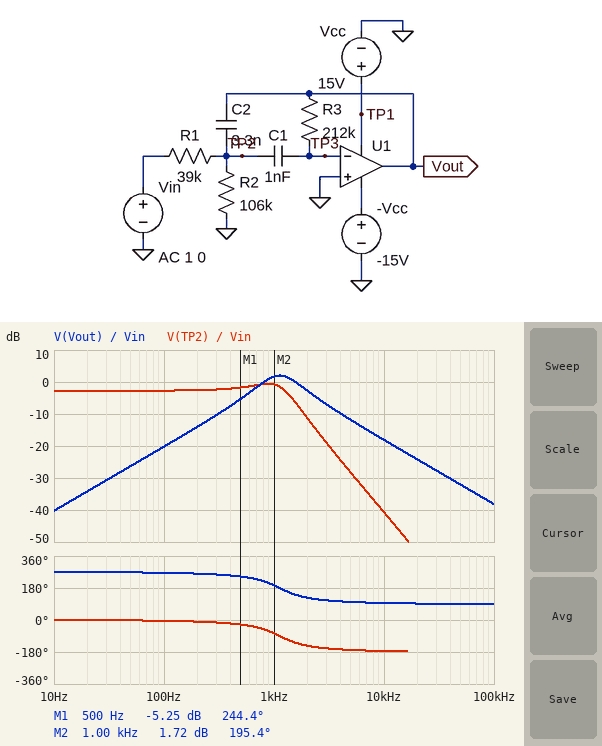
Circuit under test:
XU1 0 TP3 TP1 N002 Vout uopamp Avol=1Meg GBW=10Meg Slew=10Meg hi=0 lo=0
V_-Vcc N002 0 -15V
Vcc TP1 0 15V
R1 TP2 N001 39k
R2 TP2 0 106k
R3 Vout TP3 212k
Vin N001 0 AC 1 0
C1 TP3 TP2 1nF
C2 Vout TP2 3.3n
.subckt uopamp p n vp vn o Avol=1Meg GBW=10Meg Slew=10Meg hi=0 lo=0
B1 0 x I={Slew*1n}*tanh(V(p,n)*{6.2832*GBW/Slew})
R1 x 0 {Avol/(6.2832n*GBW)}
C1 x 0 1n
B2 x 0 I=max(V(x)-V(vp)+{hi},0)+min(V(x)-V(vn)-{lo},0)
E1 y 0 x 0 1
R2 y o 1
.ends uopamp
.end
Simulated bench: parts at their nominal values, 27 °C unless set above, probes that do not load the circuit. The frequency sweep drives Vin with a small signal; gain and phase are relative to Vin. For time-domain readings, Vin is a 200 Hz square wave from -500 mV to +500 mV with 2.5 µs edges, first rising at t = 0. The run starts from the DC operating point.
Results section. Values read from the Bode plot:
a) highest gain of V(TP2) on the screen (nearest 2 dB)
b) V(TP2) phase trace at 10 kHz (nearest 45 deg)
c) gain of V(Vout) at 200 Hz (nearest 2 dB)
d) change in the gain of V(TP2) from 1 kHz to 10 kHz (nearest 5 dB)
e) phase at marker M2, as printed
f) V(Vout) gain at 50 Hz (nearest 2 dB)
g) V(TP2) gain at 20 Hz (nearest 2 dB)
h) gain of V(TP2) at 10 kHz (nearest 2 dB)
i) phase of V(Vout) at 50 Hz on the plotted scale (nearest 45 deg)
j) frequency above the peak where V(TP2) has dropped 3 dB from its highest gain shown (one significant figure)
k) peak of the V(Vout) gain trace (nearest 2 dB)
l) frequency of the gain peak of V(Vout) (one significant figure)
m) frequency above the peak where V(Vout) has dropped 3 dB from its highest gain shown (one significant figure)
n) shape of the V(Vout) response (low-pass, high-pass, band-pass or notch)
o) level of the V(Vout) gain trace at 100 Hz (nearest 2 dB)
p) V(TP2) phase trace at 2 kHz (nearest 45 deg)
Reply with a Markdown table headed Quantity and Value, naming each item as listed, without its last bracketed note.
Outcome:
| Quantity | Value |
|---|---|
| highest gain of V(TP2) on the screen | 0 dB |
| V(TP2) phase trace at 10 kHz | -180 deg |
| gain of V(Vout) at 200 Hz | -14 dB |
| change in the gain of V(TP2) from 1 kHz to 10 kHz | -40 dB |
| phase at marker M2, as printed | 195.4 deg |
| V(Vout) gain at 50 Hz | -26 dB |
| V(TP2) gain at 20 Hz | -2 dB |
| gain of V(TP2) at 10 kHz | -40 dB |
| phase of V(Vout) at 50 Hz on the plotted scale | 270 deg |
| frequency above the peak where V(TP2) has dropped 3 dB from its highest gain shown | 1 kHz |
| peak of the V(Vout) gain trace | 2 dB |
| frequency of the gain peak of V(Vout) | 1 kHz |
| frequency above the peak where V(Vout) has dropped 3 dB from its highest gain shown | 2 kHz |
| shape of the V(Vout) response | band-pass |
| level of the V(Vout) gain trace at 100 Hz | -20 dB |
| V(TP2) phase trace at 2 kHz | -135 deg |
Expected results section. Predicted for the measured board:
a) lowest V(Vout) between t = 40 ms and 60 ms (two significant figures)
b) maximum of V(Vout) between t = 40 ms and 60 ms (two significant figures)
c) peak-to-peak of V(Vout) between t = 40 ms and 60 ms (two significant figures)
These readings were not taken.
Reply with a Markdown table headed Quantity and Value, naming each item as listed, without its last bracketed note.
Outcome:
| Quantity | Value |
|---|---|
| lowest V(Vout) between t = 40 ms and 60 ms | -640 mV |
| maximum of V(Vout) between t = 40 ms and 60 ms | 640 mV |
| peak-to-peak of V(Vout) between t = 40 ms and 60 ms | 1.3 V |
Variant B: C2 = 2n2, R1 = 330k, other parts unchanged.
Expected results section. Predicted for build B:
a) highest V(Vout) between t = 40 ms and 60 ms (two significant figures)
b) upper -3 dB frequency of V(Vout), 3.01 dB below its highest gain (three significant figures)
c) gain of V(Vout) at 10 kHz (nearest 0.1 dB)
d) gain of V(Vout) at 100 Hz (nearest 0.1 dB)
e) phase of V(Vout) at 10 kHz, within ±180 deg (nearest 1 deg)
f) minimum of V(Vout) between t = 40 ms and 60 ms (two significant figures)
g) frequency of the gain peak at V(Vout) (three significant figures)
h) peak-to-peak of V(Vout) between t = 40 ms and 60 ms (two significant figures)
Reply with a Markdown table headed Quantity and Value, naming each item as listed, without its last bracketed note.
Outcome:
| Quantity | Value |
|---|---|
| highest V(Vout) between t = 40 ms and 60 ms | 130 mV |
| upper -3 dB frequency of V(Vout), 3.01 dB below its highest gain | 1.53 kHz |
| gain of V(Vout) at 10 kHz | -33.2 dB |
| gain of V(Vout) at 100 Hz | -29.8 dB |
| phase of V(Vout) at 10 kHz, within ±180 deg | 96 deg |
| minimum of V(Vout) between t = 40 ms and 60 ms | -130 mV |
| frequency of the gain peak at V(Vout) | 823 Hz |
| peak-to-peak of V(Vout) between t = 40 ms and 60 ms | 250 mV |
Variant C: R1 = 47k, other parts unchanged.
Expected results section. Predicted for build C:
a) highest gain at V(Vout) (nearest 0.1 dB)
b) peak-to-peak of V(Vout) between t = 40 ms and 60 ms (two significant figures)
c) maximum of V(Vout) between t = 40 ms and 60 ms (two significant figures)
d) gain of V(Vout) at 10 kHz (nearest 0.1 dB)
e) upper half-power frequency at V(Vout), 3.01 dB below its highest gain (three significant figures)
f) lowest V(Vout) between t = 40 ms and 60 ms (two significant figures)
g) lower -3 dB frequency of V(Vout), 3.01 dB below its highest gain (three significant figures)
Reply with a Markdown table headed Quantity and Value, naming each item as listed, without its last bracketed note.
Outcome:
| Quantity | Value |
|---|---|
| highest gain at V(Vout) | 0.4 dB |
| peak-to-peak of V(Vout) between t = 40 ms and 60 ms | 1.1 V |
| maximum of V(Vout) between t = 40 ms and 60 ms | 550 mV |
| gain of V(Vout) at 10 kHz | -19.7 dB |
| upper half-power frequency at V(Vout), 3.01 dB below its highest gain | 1.65 kHz |
| lowest V(Vout) between t = 40 ms and 60 ms | -550 mV |
| lower -3 dB frequency of V(Vout), 3.01 dB below its highest gain | 673 Hz |
